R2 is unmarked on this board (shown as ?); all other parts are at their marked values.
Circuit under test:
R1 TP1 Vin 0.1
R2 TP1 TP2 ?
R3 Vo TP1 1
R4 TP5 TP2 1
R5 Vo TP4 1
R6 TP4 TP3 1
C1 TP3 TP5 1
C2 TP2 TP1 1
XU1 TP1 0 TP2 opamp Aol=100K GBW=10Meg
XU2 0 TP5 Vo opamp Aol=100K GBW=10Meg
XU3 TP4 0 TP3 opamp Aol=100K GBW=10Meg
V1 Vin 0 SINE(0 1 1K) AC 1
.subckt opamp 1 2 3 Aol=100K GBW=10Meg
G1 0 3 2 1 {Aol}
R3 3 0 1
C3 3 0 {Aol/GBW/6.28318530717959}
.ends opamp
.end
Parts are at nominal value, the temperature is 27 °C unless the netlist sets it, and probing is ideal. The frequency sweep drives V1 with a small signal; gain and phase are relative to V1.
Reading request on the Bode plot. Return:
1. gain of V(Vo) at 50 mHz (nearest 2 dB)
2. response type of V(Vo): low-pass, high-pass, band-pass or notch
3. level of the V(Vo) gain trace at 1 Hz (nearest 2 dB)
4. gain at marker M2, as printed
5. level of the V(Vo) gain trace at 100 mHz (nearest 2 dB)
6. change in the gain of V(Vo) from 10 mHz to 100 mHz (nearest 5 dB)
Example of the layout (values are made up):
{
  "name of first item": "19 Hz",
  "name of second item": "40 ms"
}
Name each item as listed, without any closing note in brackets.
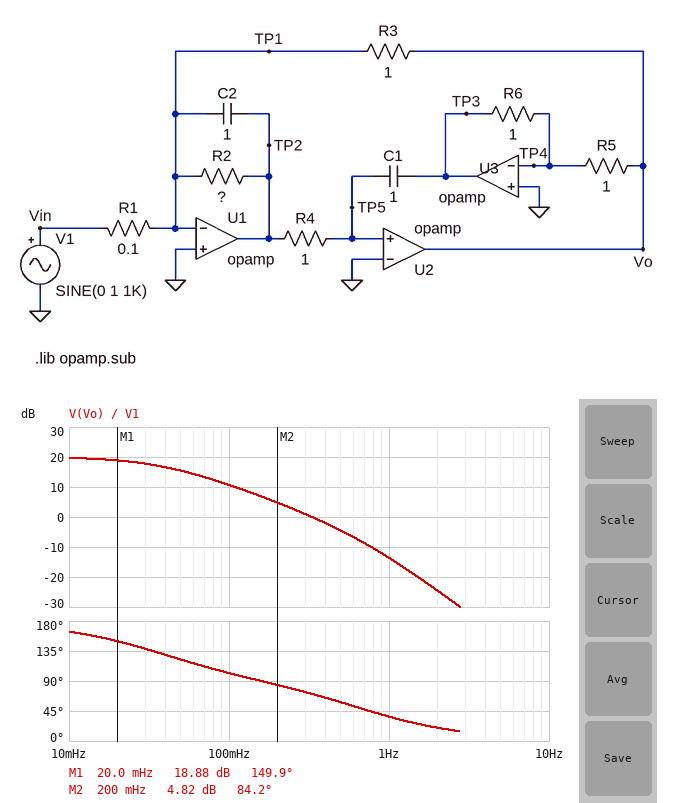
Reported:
{
  "gain of V(Vo) at 50 mHz": "16 dB",
  "response type of V(Vo): low-pass, high-pass, band-pass or notch": "low-pass",
  "level of the V(Vo) gain trace at 1 Hz": "-14 dB",
  "gain at marker M2, as printed": "4.82 dB",
  "level of the V(Vo) gain trace at 100 mHz": "10 dB",
  "change in the gain of V(Vo) from 10 mHz to 100 mHz": "-10 dB"
}
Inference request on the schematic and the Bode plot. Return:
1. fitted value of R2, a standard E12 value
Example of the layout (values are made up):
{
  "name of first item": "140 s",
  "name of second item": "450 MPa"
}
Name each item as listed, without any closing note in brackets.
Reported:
{
  "fitted value of R2, a standard E12 value": "0.22 Ω"
}
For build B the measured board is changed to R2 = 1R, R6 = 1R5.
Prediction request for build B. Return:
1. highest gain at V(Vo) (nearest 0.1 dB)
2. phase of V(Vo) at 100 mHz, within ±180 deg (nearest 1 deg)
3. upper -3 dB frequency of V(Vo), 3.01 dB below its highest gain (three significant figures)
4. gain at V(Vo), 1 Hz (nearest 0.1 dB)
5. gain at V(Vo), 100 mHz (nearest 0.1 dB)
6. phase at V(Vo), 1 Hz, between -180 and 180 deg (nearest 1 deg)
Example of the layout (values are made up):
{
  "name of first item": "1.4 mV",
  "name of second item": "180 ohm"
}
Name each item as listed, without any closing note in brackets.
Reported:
{
  "highest gain at V(Vo)": "20.3 dB",
  "phase of V(Vo) at 100 mHz, within ±180 deg": "113 deg",
  "upper -3 dB frequency of V(Vo), 3.01 dB below its highest gain": "143 mHz",
  "gain at V(Vo), 1 Hz": "-15.4 dB",
  "gain at V(Vo), 100 mHz": "19.8 dB",
  "phase at V(Vo), 1 Hz, between -180 and 180 deg": "9 deg"
}
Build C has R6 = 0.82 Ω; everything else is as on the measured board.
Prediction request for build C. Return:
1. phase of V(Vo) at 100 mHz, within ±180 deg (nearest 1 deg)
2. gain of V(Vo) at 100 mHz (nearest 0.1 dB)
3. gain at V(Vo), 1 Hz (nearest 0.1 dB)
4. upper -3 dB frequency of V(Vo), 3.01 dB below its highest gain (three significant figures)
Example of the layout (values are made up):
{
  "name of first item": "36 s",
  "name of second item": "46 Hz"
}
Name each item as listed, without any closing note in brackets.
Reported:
{
  "phase of V(Vo) at 100 mHz, within ±180 deg": "106 deg",
  "gain of V(Vo) at 100 mHz": "12.3 dB",
  "gain at V(Vo), 1 Hz": "-11.9 dB",
  "upper -3 dB frequency of V(Vo), 3.01 dB below its highest gain": "45.4 mHz"
}
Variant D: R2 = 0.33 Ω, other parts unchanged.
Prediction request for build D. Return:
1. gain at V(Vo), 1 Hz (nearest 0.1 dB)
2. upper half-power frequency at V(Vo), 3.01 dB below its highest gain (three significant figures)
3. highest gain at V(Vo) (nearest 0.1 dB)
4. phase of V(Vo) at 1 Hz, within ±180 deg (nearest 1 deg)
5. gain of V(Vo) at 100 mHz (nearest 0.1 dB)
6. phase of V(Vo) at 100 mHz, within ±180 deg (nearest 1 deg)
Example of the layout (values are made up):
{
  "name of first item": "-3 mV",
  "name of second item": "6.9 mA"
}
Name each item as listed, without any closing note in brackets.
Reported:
{
  "gain at V(Vo), 1 Hz": "-12.7 dB",
  "upper half-power frequency at V(Vo), 3.01 dB below its highest gain": "58.8 mHz",
  "highest gain at V(Vo)": "20.0 dB",
  "phase of V(Vo) at 1 Hz, within ±180 deg": "26 deg",
  "gain of V(Vo) at 100 mHz": "14.0 dB",
  "phase of V(Vo) at 100 mHz, within ±180 deg": "108 deg"
}
